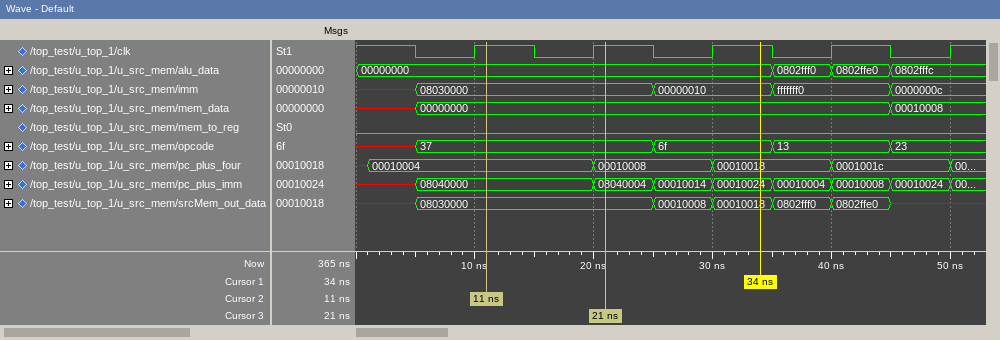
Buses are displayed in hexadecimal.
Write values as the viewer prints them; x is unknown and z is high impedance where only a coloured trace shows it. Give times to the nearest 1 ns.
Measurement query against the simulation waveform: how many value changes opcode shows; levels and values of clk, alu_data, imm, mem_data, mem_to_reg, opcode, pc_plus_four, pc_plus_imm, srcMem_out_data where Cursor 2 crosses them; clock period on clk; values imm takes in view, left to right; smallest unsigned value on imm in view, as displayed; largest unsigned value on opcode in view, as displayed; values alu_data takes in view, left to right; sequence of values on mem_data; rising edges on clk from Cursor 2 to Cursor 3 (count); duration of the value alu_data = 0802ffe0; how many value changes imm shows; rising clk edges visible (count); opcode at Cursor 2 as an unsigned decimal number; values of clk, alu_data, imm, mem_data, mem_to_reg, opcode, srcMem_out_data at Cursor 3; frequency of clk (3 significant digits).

4
clk=1, alu_data=00000000, imm=08030000, mem_data=00000000, mem_to_reg=0, opcode=37, pc_plus_four=00010004, pc_plus_imm=08040000, srcMem_out_data=08030000
10 ns
x, 08030000, 00000010, fffffff0, 0000000c
0000000c
6f
00000000, 0802fff0, 0802ffe0, 0802fffc
x, 00000000, 00010008
1
5 ns
4
5
55
clk=1, alu_data=00000000, imm=08030000, mem_data=00000000, mem_to_reg=0, opcode=37, srcMem_out_data=08030000
100 MHz
